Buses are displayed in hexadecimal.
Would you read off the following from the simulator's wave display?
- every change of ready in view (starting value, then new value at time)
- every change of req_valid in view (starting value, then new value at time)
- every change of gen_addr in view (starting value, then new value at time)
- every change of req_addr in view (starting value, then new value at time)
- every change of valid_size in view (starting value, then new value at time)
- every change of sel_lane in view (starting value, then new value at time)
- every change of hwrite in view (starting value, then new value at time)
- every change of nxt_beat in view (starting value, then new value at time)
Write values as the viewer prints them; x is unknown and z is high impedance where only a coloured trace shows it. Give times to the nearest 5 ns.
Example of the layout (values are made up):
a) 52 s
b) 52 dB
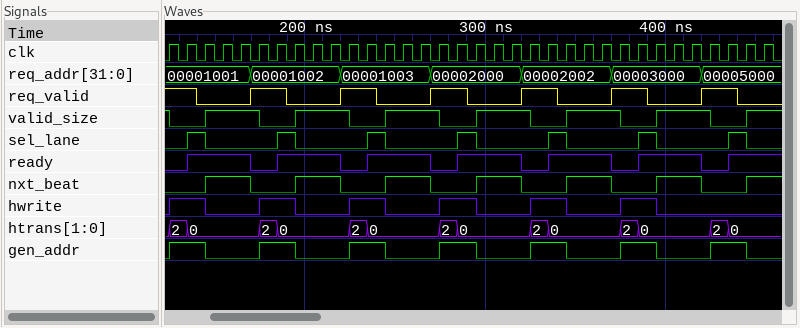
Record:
a) 0, 1 at 135 ns, 0 at 170 ns, 1 at 185 ns, 0 at 220 ns, 1 at 235 ns, 0 at 270 ns, 1 at 285 ns, 0 at 320 ns, 1 at 335 ns, 0 at 370 ns, 1 at 385 ns, 0 at 420 ns, 1 at 435 ns
b) 1, 0 at 140 ns, 1 at 170 ns, 0 at 190 ns, 1 at 220 ns, 0 at 240 ns, 1 at 270 ns, 0 at 290 ns, 1 at 320 ns, 0 at 340 ns, 1 at 370 ns, 0 at 390 ns, 1 at 420 ns, 0 at 440 ns
c) 0, 1 at 125 ns, 0 at 145 ns, 1 at 175 ns, 0 at 195 ns, 1 at 225 ns, 0 at 245 ns, 1 at 275 ns, 0 at 295 ns, 1 at 325 ns, 0 at 345 ns, 1 at 375 ns, 0 at 395 ns, 1 at 425 ns, 0 at 445 ns
d) 00001001, 00001002 at 170 ns, 00001003 at 220 ns, 00002000 at 270 ns, 00002002 at 320 ns, 00003000 at 370 ns, 00005000 at 420 ns
e) 1, 0 at 125 ns, 1 at 145 ns, 0 at 175 ns, 1 at 195 ns, 0 at 225 ns, 1 at 245 ns, 0 at 275 ns, 1 at 295 ns, 0 at 325 ns, 1 at 345 ns, 0 at 375 ns, 1 at 395 ns, 0 at 425 ns, 1 at 445 ns
f) 0, 1 at 135 ns, 0 at 145 ns, 1 at 185 ns, 0 at 195 ns, 1 at 235 ns, 0 at 245 ns, 1 at 285 ns, 0 at 295 ns, 1 at 335 ns, 0 at 345 ns, 1 at 385 ns, 0 at 395 ns, 1 at 435 ns, 0 at 445 ns
g) 0, 1 at 125 ns, 0 at 145 ns, 1 at 175 ns, 0 at 195 ns, 1 at 225 ns, 0 at 245 ns, 1 at 275 ns, 0 at 295 ns, 1 at 325 ns, 0 at 345 ns, 1 at 375 ns, 0 at 395 ns
h) 0, 1 at 145 ns, 0 at 170 ns, 1 at 195 ns, 0 at 220 ns, 1 at 245 ns, 0 at 270 ns, 1 at 295 ns, 0 at 320 ns, 1 at 345 ns, 0 at 370 ns, 1 at 395 ns, 0 at 420 ns, 1 at 445 ns
